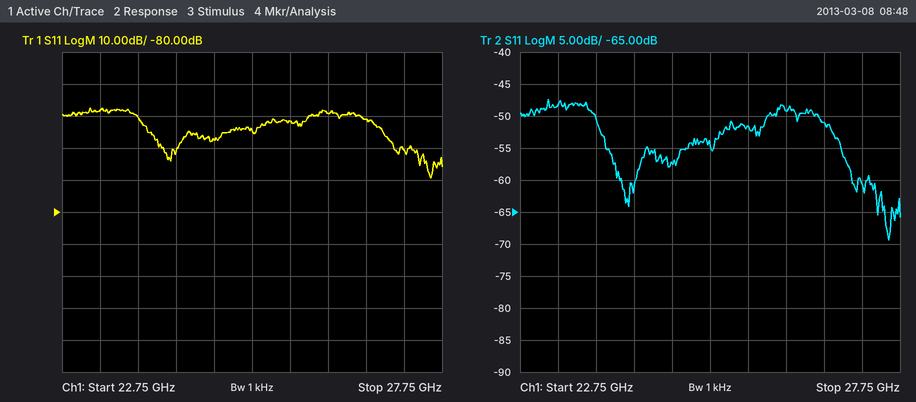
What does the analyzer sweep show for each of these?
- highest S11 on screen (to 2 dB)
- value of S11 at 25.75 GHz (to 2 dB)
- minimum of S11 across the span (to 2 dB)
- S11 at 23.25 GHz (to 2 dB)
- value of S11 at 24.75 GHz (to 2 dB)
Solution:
-48 dB
-52 dB
-70 dB
-48 dB
-58 dB
